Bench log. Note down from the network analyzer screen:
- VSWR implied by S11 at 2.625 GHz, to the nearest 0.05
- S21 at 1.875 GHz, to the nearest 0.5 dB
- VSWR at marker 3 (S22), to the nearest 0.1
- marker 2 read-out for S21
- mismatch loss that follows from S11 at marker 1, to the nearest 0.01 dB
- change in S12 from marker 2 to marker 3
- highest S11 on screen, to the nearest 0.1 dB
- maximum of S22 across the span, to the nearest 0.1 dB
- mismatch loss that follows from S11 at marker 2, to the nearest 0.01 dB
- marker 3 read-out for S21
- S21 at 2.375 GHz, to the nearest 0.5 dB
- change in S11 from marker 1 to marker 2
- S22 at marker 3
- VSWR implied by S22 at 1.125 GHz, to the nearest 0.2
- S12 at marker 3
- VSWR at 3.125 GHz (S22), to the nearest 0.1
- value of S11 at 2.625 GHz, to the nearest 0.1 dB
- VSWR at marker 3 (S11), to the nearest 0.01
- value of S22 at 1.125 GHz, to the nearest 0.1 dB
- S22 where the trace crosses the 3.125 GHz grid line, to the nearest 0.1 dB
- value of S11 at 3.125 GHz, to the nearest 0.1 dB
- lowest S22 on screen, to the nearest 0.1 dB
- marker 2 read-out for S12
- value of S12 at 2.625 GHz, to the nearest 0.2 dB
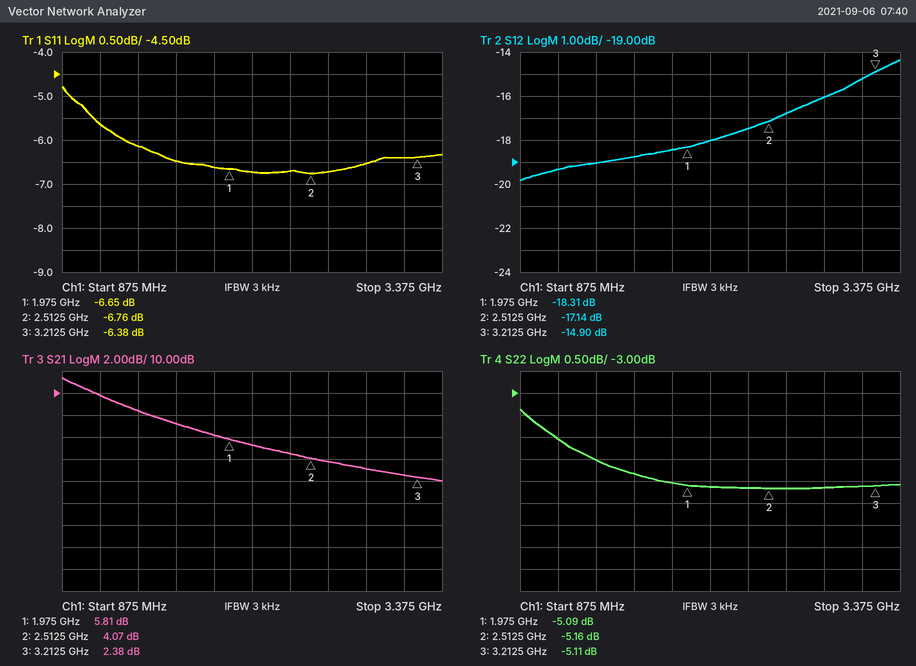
2.70
6.0 dB
3.5
4.07 dB
1.06 dB
2.24 dB
-4.8 dB
-3.4 dB
1.03 dB
2.38 dB
4.5 dB
-0.11 dB
-5.11 dB
4.4
-14.90 dB
3.5
-6.7 dB
2.84
-4.0 dB
-5.1 dB
-6.4 dB
-5.2 dB
-17.14 dB
-16.8 dB
